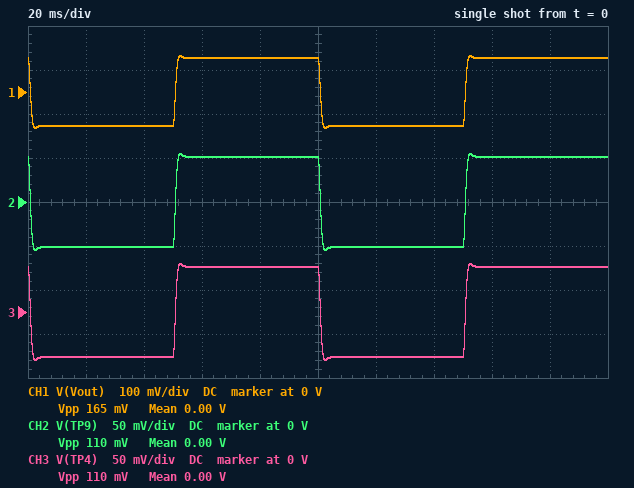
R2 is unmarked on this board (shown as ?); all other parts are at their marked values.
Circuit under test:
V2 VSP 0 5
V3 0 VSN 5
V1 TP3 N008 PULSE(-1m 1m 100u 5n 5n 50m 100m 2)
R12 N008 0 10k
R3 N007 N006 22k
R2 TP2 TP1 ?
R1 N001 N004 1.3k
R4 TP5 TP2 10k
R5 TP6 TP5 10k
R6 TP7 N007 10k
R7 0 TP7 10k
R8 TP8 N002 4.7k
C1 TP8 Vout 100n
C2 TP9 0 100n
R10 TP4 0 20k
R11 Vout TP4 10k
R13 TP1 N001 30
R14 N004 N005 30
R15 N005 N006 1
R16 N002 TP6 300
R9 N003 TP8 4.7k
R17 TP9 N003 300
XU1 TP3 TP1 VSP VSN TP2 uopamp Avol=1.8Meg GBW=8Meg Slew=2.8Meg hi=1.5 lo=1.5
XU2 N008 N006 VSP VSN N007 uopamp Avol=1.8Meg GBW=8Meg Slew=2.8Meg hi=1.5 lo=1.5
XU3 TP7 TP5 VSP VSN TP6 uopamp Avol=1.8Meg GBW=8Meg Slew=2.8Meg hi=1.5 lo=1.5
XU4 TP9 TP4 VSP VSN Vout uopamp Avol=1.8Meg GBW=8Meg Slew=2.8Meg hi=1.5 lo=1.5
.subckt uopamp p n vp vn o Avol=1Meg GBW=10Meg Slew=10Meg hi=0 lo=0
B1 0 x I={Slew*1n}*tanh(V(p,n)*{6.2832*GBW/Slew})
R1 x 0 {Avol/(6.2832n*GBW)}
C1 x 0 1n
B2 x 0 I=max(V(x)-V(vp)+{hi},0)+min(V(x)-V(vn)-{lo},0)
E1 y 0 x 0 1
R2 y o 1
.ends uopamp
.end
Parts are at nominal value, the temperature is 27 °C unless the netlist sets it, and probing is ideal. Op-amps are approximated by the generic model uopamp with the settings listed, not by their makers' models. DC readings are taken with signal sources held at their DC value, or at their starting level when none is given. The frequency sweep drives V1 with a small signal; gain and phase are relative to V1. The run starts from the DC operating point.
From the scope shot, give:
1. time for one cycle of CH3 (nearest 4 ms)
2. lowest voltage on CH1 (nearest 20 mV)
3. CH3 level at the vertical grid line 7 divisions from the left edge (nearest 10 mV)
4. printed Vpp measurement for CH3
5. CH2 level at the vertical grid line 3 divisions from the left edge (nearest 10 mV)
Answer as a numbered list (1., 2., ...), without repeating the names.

1. 100 ms
2. -80 mV
3. -50 mV
4. 110 mV
5. 50 mV
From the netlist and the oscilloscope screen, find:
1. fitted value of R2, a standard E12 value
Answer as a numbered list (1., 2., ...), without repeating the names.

1. 47 kΩ
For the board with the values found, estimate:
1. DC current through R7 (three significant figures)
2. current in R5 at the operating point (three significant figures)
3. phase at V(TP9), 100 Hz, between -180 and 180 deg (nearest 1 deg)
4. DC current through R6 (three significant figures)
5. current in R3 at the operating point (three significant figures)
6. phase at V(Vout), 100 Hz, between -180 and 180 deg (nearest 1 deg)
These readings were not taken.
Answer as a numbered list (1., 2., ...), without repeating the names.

1. 808 nA
2. 4.36 µA
3. 152 deg
4. 808 nA
5. 735 nA
6. 152 deg
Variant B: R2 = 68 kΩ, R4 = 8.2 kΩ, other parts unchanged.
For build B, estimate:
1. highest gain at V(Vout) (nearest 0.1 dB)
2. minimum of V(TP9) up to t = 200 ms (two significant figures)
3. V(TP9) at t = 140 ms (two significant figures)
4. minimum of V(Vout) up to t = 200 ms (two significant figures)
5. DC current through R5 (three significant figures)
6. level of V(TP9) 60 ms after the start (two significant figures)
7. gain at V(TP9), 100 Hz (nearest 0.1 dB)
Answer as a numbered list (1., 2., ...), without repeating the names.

1. 41.6 dB
2. -85 mV
3. -80 mV
4. -130 mV
5. 7.20 µA
6. 80 mV
7. 37.9 dB
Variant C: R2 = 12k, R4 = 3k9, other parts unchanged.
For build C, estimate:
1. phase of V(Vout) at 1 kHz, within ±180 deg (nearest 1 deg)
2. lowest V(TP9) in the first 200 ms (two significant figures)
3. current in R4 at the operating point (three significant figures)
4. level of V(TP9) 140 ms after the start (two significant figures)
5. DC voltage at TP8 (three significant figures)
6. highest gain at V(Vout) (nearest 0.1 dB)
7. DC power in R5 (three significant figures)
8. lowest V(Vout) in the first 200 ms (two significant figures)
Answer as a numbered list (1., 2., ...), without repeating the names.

1. 28 deg
2. -57 mV
3. 4.59 µA
4. -54 mV
5. 54.0 mV
6. 38.2 dB
7. 211 nW
8. -86 mV
